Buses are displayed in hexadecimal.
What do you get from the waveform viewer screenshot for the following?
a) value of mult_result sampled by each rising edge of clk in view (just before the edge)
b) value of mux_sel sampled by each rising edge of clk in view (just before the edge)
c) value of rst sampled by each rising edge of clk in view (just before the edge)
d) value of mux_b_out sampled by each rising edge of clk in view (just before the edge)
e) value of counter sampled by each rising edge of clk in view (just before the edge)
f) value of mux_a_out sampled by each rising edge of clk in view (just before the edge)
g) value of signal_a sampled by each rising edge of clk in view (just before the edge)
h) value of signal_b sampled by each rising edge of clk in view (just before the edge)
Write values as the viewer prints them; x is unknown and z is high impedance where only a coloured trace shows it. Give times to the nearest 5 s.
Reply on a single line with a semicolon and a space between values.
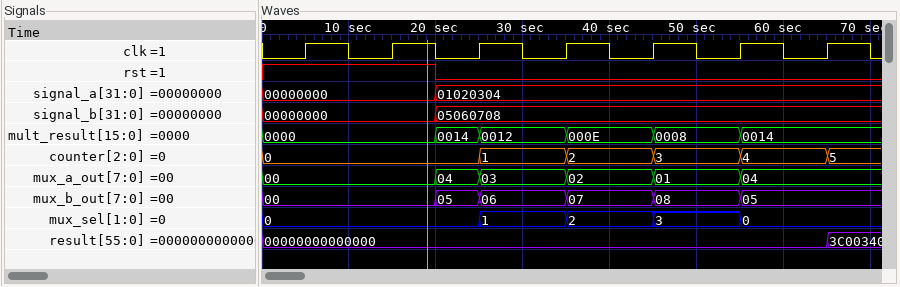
0000, 0000, 0014, 0012, 000E, 0008, 0014; 0, 0, 0, 1, 2, 3, 0; 1 1 0 0 0 0 0; 00, 00, 05, 06, 07, 08, 05; 0, 0, 0, 1, 2, 3, 4; 00, 00, 04, 03, 02, 01, 04; 00000000, 00000000, 01020304, 01020304, 01020304, 01020304, 01020304; 00000000, 00000000, 05060708, 05060708, 05060708, 05060708, 05060708
